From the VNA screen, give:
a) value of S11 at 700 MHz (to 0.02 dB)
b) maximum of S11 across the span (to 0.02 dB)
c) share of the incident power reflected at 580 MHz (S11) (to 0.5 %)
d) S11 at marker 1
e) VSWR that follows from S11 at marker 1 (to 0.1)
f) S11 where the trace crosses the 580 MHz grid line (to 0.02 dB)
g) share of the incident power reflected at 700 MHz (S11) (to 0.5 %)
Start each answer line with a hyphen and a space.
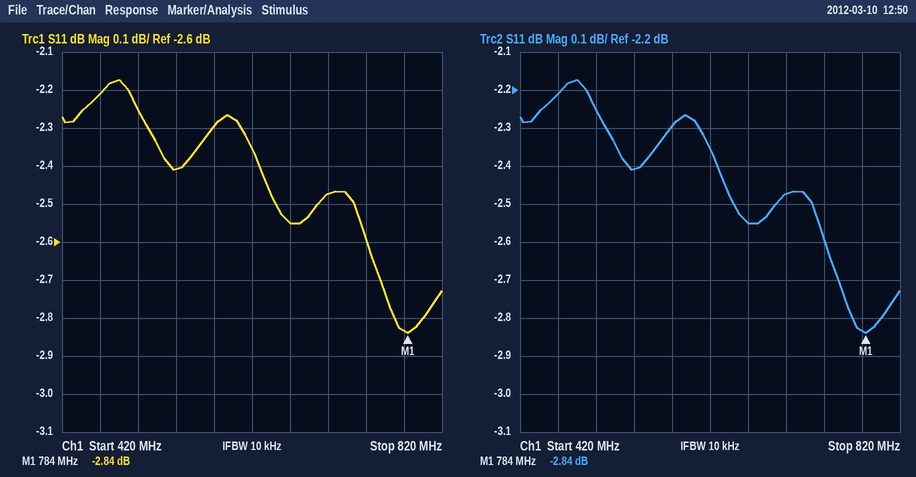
- -2.48 dB
- -2.18 dB
- 59.0 %
- -2.84 dB
- 6.2
- -2.30 dB
- 56.5 %
